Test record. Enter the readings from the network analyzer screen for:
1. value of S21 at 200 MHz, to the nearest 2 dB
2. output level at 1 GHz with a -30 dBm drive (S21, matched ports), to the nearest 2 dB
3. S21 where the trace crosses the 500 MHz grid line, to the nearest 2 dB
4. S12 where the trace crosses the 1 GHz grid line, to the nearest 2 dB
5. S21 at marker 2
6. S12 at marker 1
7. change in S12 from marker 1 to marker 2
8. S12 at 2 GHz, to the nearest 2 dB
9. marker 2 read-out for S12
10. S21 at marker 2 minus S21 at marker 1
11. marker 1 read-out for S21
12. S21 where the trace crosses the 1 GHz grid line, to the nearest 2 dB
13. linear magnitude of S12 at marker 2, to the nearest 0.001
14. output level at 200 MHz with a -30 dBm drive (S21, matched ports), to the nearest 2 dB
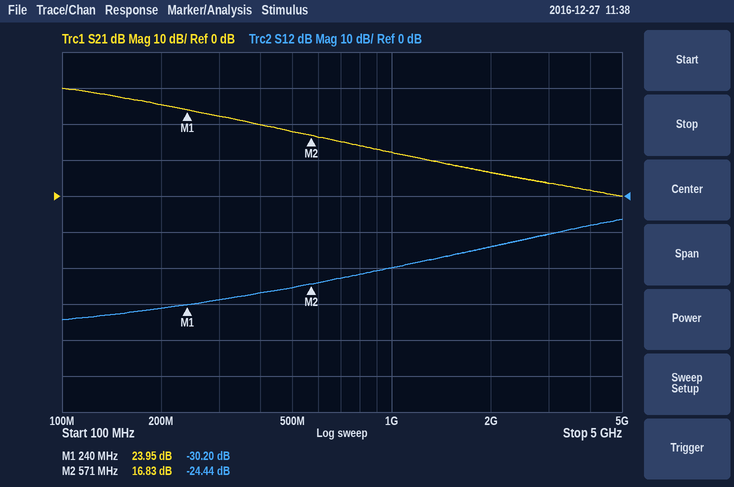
26 dB
-18 dBm
18 dB
-20 dB
16.83 dB
-30.20 dB
5.76 dB
-14 dB
-24.44 dB
-7.12 dB
23.95 dB
12 dB
0.060
-4 dBm
